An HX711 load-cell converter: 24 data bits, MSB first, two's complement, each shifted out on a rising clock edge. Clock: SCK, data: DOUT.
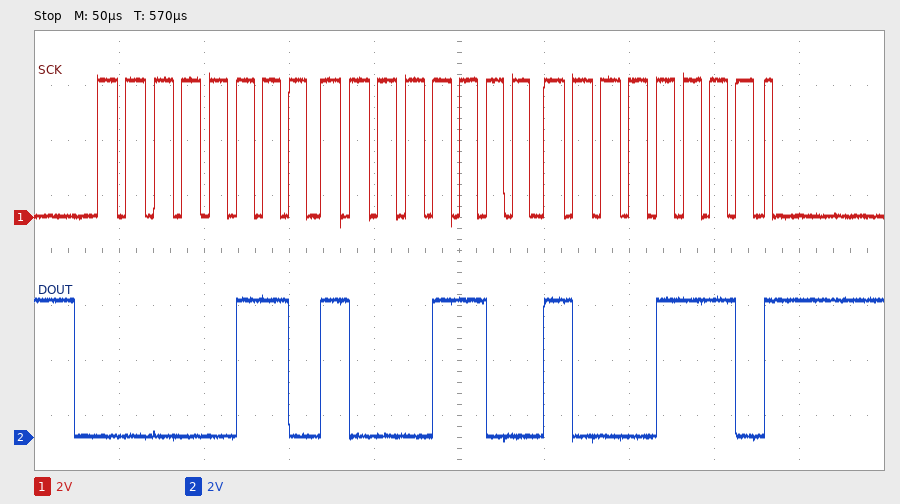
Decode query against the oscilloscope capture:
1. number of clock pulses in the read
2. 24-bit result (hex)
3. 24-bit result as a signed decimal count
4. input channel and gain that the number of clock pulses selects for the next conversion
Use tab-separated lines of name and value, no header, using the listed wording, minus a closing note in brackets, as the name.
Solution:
number of clock pulses in the read	25
24-bit result	0x068C8E
24-bit result as a signed decimal count	429198
input channel and gain that the number of clock pulses selects for the next conversion	channel A, gain 128
